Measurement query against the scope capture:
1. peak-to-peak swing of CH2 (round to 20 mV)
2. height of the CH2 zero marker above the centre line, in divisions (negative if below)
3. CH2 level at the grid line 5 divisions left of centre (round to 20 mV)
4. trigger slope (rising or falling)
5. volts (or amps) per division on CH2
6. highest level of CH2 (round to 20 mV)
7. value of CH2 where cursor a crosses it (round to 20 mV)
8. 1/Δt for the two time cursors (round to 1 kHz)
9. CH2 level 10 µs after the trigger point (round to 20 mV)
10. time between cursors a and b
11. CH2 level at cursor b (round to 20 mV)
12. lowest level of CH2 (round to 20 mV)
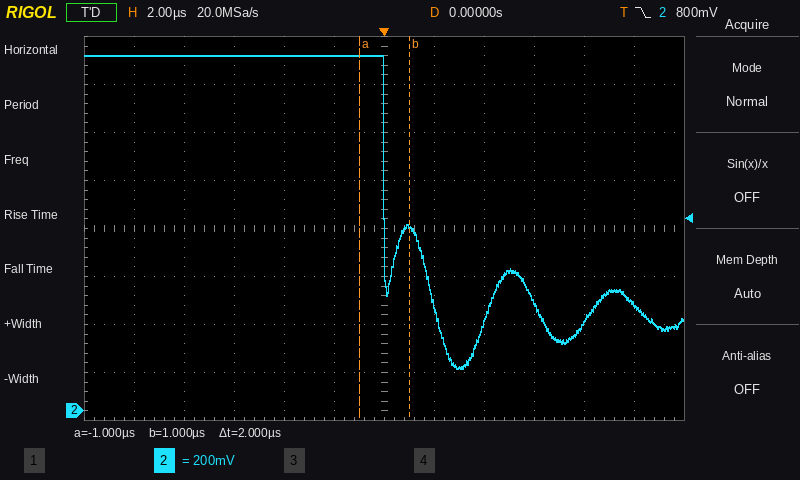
1.30 V
-3.8 div
1.48 V
falling
200 mV
1.48 V
1.48 V
500 kHz
440 mV
2 µs
760 mV
180 mV
